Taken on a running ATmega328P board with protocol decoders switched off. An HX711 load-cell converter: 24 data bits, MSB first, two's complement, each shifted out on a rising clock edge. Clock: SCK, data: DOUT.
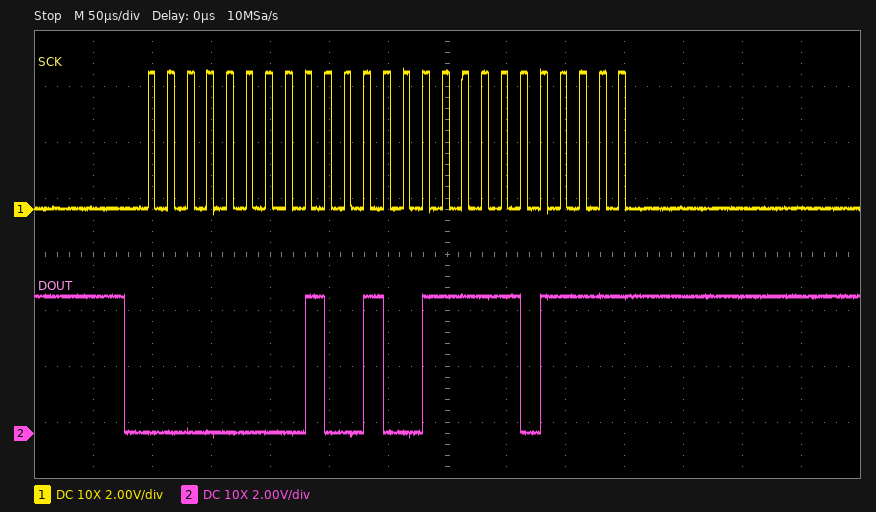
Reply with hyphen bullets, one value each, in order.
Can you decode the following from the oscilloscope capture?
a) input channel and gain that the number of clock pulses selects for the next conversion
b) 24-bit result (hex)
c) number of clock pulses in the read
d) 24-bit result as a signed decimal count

- channel A, gain 128
- 0x0093EF
- 25
- 37871
